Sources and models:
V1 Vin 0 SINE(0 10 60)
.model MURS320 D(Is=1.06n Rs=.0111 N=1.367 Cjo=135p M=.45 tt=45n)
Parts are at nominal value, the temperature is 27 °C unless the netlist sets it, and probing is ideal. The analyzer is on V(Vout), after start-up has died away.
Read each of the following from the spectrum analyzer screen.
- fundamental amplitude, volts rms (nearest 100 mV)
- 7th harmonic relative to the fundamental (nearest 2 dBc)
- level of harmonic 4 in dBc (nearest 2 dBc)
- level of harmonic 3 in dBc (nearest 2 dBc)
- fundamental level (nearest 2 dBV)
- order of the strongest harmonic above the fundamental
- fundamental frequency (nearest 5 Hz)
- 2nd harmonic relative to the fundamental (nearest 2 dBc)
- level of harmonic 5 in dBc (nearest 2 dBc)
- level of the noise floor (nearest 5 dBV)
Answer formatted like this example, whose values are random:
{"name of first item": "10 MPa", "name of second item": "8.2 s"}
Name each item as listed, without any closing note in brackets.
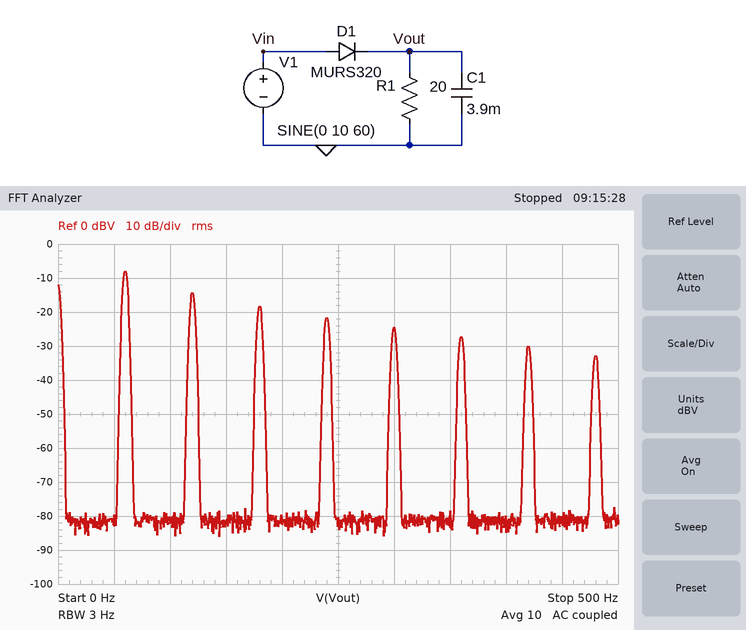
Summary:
{"fundamental amplitude, volts rms": "400 mV", "7th harmonic relative to the fundamental": "-22 dBc", "level of harmonic 4 in dBc": "-14 dBc", "level of harmonic 3 in dBc": "-10 dBc", "fundamental level": "-8 dBV", "order of the strongest harmonic above the fundamental": "2", "fundamental frequency": "60 Hz", "2nd harmonic relative to the fundamental": "-6 dBc", "level of harmonic 5 in dBc": "-16 dBc", "level of the noise floor": "-80 dBV"}
